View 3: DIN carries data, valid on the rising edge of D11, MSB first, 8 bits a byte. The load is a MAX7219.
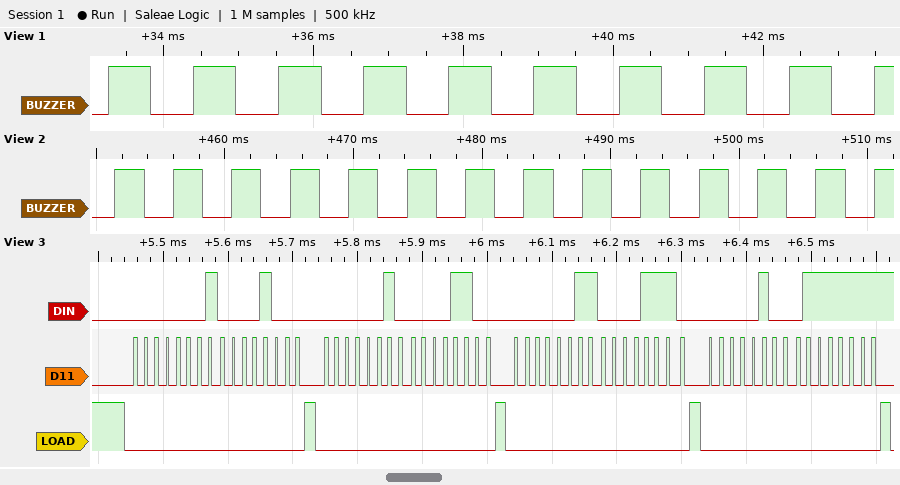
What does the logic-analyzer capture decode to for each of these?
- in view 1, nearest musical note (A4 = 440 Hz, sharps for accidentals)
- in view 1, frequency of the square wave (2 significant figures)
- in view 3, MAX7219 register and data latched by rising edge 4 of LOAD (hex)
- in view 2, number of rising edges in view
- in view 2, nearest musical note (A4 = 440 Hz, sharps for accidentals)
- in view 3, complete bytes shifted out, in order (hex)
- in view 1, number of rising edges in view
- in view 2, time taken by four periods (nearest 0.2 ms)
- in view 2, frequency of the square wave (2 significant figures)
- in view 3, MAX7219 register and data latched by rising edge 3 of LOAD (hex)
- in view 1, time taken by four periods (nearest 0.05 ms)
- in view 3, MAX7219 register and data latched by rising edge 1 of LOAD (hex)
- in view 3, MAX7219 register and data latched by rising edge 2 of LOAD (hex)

A5
880 Hz
register 0x4, data 0x7F
14
A3
0x01 0x08 0x02 0x0C 0x03 0x0E 0x04 0x7F
10
18.2 ms
220 Hz
register 0x3, data 0x0E
4.55 ms
register 0x1, data 0x08
register 0x2, data 0x0C
